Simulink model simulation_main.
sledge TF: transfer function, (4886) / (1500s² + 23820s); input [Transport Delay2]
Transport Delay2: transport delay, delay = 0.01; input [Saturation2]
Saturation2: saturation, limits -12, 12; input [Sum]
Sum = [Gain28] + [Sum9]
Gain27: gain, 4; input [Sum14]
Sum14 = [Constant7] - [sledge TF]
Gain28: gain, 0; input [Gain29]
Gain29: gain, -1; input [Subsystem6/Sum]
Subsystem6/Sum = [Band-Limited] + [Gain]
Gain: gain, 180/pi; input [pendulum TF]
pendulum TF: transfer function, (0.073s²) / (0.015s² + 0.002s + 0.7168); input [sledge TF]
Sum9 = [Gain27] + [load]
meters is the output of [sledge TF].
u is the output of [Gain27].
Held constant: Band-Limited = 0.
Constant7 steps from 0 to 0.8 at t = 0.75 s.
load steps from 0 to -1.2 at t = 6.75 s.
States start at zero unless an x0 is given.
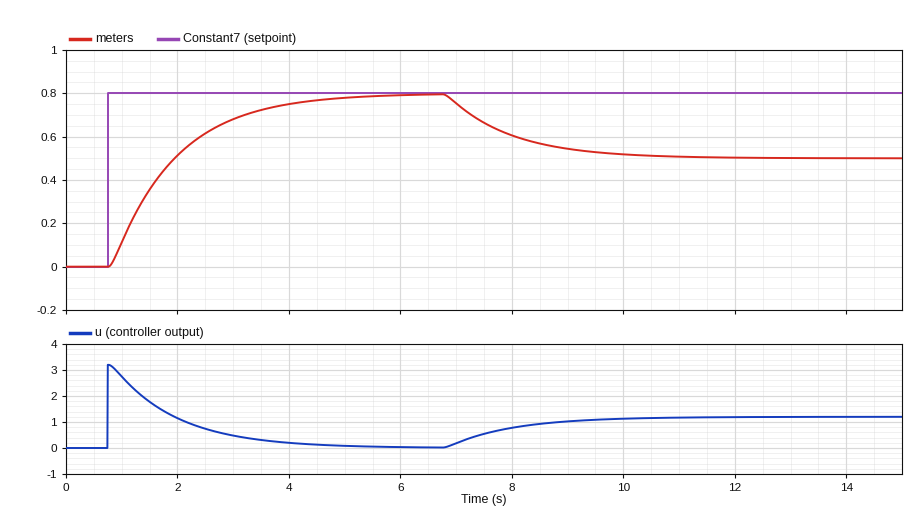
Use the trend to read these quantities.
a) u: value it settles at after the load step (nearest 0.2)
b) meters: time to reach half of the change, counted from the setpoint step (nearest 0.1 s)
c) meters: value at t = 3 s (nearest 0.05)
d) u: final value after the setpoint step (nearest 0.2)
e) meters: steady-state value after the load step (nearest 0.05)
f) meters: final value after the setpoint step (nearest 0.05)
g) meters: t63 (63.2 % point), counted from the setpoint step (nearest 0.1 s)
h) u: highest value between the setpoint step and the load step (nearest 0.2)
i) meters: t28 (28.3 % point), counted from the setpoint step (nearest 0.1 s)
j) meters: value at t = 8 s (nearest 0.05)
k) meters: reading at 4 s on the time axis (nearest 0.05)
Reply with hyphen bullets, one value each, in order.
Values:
- 1.2
- 0.9 s
- 0.70
- 0.0
- 0.50
- 0.80
- 1.2 s
- 3.2
- 0.5 s
- 0.60
- 0.75
